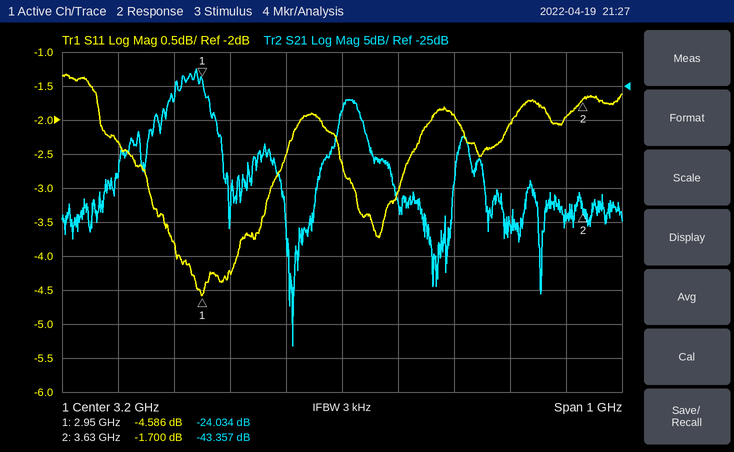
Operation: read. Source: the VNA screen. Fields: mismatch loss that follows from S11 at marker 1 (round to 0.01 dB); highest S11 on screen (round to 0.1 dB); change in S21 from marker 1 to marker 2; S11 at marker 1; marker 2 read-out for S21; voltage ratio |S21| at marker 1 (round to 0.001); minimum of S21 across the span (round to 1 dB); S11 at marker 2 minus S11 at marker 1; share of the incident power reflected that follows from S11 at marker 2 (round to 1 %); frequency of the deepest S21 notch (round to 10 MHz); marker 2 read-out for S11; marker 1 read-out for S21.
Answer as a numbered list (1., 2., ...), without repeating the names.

1. 1.86 dB
2. -1.3 dB
3. -19.323 dB
4. -4.586 dB
5. -43.357 dB
6. 0.063
7. -63 dB
8. 2.886 dB
9. 68 %
10. 3.11 GHz
11. -1.700 dB
12. -24.034 dB
